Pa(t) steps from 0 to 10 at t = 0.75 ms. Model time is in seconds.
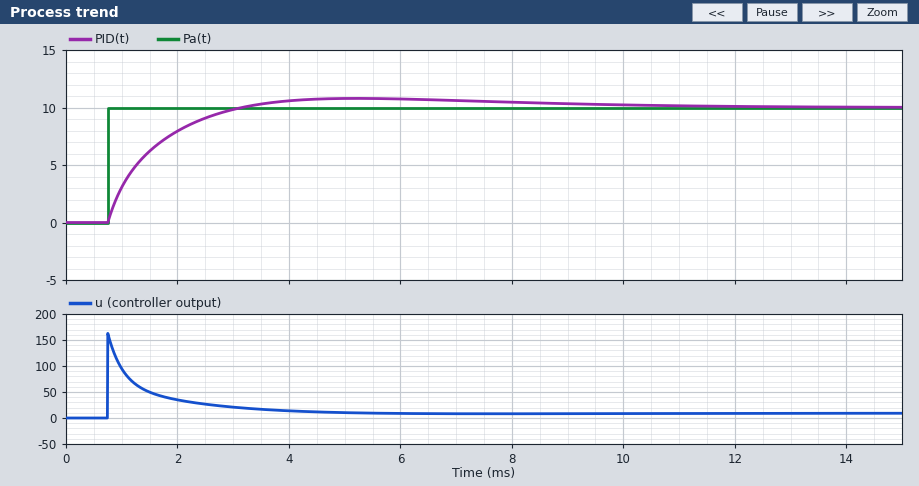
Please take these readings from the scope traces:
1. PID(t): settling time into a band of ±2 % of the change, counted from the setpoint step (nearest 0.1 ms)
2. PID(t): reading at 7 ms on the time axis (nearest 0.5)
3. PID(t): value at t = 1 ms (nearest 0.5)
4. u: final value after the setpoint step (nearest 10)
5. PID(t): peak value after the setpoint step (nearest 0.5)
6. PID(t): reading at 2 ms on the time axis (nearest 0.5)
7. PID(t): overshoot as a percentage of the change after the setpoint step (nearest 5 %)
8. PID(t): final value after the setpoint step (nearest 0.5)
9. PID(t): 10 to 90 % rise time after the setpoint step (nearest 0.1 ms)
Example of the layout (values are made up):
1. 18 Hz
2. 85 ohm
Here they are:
1. 9.6 ms
2. 10.5
3. 3.0
4. 10
5. 11.0
6. 8.0
7. 10 %
8. 10.0
9. 1.6 ms
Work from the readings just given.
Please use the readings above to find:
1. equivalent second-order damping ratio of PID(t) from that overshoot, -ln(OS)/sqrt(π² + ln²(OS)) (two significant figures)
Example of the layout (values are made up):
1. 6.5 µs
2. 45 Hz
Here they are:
1. 0.59
